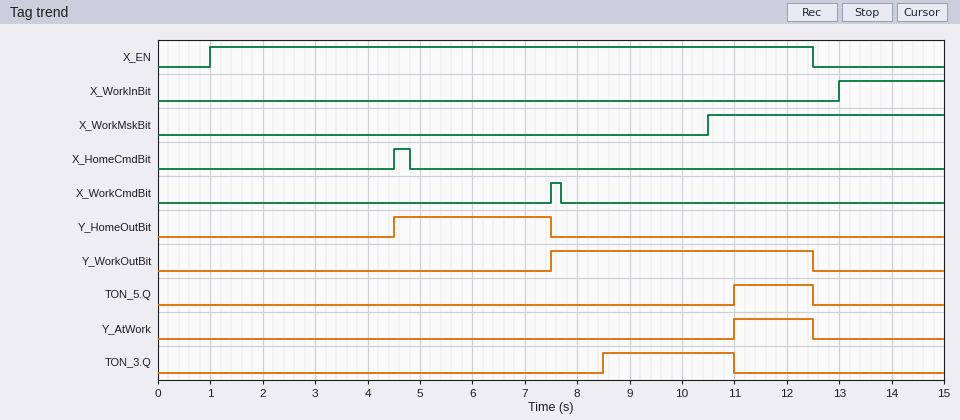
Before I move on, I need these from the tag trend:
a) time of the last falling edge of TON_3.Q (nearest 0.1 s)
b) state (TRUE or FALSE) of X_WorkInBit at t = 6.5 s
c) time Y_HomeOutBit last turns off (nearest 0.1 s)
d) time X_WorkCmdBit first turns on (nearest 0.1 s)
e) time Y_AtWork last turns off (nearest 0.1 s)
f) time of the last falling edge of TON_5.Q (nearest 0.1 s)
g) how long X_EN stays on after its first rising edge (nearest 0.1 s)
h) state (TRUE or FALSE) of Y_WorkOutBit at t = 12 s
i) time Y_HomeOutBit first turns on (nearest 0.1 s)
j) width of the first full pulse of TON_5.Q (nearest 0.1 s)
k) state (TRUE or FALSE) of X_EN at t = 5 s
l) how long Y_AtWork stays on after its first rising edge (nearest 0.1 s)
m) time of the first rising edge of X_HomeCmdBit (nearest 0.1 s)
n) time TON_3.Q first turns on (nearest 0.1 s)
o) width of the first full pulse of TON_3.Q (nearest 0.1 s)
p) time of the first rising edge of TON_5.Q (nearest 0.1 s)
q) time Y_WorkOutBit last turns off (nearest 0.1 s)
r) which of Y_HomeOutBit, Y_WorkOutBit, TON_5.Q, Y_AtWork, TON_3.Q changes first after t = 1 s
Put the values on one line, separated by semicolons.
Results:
11.0 s; FALSE; 7.5 s; 7.5 s; 12.5 s; 12.5 s; 11.5 s; TRUE; 4.5 s; 1.5 s; TRUE; 1.5 s; 4.5 s; 8.5 s; 2.5 s; 11.0 s; 12.5 s; Y_HomeOutBit
